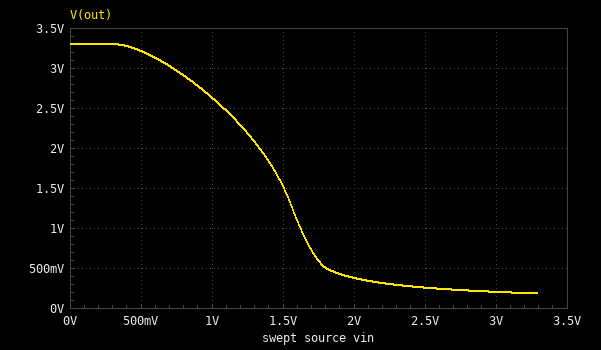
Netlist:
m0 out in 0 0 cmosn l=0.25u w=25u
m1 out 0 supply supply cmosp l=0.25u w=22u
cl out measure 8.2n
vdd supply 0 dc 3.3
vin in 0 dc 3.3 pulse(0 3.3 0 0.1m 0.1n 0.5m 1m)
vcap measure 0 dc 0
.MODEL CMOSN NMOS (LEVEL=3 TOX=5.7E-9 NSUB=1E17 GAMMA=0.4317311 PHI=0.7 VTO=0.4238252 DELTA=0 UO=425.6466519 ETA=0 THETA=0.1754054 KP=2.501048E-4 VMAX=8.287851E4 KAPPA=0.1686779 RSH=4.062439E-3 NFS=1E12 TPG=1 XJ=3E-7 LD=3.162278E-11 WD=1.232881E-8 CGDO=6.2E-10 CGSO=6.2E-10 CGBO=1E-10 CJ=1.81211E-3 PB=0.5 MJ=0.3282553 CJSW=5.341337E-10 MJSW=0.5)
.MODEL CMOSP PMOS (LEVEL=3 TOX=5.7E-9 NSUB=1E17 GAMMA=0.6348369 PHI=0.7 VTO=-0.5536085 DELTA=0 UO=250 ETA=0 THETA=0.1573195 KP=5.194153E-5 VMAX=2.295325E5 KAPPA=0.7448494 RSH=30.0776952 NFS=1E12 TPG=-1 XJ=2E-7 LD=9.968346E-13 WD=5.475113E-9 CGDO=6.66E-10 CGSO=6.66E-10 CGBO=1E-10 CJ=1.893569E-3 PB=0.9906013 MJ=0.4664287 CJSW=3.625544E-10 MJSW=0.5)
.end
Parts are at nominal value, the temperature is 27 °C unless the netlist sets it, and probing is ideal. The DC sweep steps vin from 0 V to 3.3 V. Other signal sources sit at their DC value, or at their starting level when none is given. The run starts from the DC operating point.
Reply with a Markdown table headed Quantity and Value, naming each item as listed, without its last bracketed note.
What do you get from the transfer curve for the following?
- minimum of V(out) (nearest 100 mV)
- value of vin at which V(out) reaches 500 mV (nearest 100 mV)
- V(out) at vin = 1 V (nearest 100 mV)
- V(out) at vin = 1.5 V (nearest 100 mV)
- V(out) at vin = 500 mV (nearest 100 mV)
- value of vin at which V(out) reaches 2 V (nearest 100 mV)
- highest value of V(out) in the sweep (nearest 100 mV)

| Quantity | Value |
|---|---|
| minimum of V(out) | 200 mV |
| value of vin at which V(out) reaches 500 mV | 1.8 V |
| V(out) at vin = 1 V | 2.6 V |
| V(out) at vin = 1.5 V | 1.5 V |
| V(out) at vin = 500 mV | 3.2 V |
| value of vin at which V(out) reaches 2 V | 1.3 V |
| highest value of V(out) in the sweep | 3.3 V |
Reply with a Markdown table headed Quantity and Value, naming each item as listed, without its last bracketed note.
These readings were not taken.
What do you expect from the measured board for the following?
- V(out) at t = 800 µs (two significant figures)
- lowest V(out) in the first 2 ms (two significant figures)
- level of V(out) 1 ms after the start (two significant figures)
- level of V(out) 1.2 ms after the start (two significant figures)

| Quantity | Value |
|---|---|
| V(out) at t = 800 µs | 3.3 V |
| lowest V(out) in the first 2 ms | 180 mV |
| level of V(out) 1 ms after the start | 3.3 V |
| level of V(out) 1.2 ms after the start | 180 mV |
